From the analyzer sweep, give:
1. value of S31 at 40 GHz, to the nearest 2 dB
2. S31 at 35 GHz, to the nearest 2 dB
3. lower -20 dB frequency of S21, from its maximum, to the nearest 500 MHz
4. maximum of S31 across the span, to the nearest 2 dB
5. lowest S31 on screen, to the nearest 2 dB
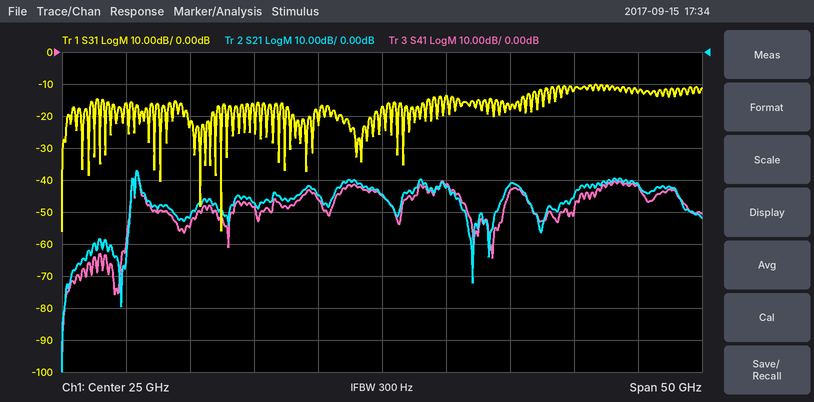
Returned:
-12 dB
-18 dB
5.0 GHz
-10 dB
-56 dB
